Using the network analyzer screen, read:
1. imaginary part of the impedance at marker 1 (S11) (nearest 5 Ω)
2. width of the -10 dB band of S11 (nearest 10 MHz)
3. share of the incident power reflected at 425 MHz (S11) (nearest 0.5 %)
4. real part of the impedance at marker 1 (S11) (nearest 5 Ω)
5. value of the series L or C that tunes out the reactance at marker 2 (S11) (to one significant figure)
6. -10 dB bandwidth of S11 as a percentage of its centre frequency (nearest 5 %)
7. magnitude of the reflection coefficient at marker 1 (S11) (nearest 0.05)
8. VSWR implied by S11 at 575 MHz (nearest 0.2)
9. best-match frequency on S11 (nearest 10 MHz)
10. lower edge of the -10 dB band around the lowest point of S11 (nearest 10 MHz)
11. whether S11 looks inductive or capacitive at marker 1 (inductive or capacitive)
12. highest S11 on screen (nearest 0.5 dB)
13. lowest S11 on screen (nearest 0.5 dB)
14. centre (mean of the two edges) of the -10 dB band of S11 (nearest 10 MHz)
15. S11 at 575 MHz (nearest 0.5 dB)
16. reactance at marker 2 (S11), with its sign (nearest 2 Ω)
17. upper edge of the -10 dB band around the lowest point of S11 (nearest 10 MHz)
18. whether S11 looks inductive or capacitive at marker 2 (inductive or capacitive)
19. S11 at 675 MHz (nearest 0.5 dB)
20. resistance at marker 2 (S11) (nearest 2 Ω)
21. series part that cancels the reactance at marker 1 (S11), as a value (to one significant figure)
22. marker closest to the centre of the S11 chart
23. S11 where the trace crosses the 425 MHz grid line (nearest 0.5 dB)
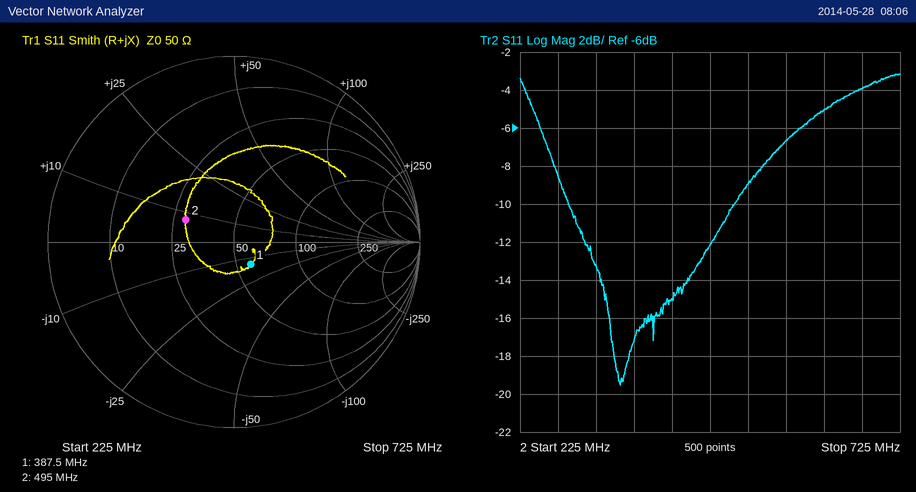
-15 Ω
220 MHz
3.0 %
60 Ω
40 pF
55 %
0.15
2.8
360 MHz
290 MHz
capacitive
-3.0 dB
-19.5 dB
400 MHz
-6.5 dB
+8 Ω
510 MHz
inductive
-4.0 dB
28 Ω
6 nH
marker 1
-15.0 dB
